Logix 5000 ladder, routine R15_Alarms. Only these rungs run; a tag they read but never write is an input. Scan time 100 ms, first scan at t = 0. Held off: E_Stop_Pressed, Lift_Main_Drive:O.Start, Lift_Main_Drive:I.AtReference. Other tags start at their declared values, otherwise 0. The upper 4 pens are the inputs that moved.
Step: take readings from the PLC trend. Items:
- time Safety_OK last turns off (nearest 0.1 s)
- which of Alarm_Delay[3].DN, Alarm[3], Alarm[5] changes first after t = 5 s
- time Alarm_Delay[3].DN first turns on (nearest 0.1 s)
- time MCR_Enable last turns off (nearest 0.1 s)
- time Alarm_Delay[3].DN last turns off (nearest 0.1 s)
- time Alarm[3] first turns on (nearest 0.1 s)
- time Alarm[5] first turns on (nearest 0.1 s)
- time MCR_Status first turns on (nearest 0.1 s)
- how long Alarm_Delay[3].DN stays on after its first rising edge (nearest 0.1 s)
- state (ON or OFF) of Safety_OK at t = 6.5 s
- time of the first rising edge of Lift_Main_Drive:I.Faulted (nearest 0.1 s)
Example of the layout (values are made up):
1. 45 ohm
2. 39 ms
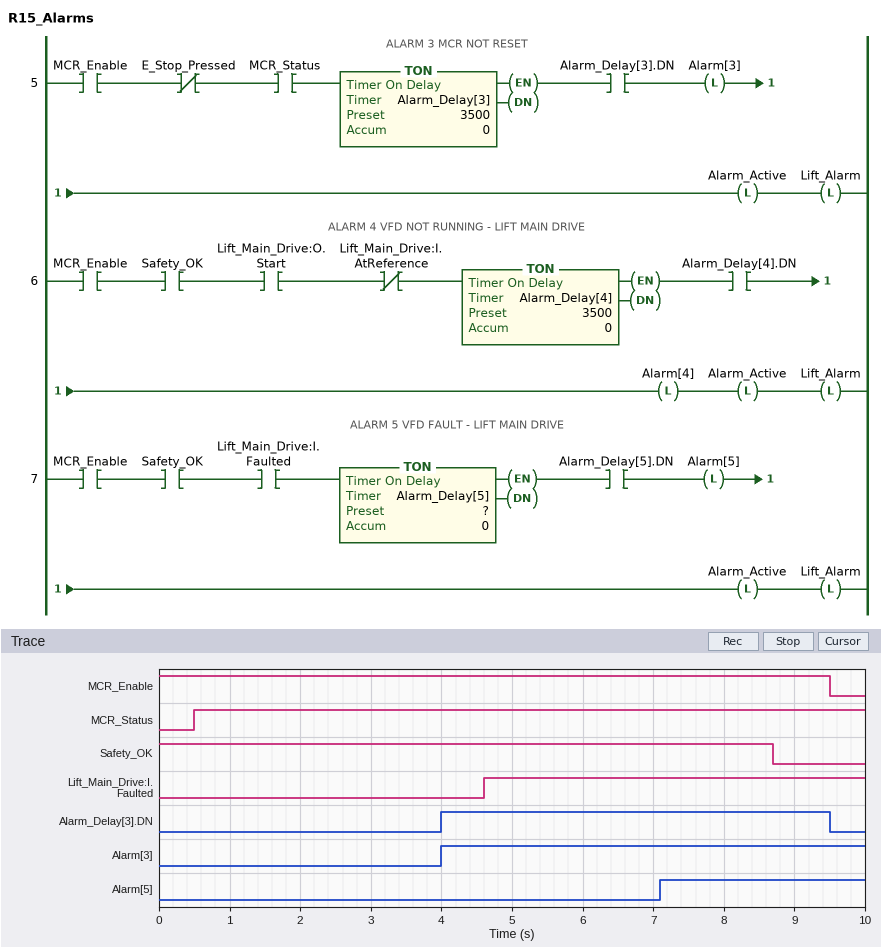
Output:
1. 8.7 s
2. Alarm[5]
3. 4.0 s
4. 9.5 s
5. 9.5 s
6. 4.0 s
7. 7.1 s
8. 0.5 s
9. 5.5 s
10. ON
11. 4.6 s
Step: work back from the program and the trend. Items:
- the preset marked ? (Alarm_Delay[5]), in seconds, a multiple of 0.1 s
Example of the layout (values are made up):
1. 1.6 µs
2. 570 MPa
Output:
1. 2.5 s
